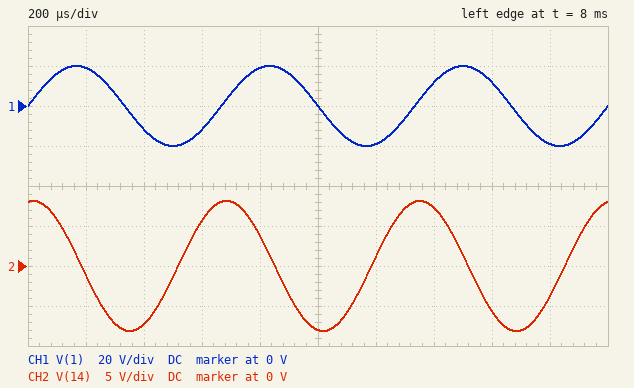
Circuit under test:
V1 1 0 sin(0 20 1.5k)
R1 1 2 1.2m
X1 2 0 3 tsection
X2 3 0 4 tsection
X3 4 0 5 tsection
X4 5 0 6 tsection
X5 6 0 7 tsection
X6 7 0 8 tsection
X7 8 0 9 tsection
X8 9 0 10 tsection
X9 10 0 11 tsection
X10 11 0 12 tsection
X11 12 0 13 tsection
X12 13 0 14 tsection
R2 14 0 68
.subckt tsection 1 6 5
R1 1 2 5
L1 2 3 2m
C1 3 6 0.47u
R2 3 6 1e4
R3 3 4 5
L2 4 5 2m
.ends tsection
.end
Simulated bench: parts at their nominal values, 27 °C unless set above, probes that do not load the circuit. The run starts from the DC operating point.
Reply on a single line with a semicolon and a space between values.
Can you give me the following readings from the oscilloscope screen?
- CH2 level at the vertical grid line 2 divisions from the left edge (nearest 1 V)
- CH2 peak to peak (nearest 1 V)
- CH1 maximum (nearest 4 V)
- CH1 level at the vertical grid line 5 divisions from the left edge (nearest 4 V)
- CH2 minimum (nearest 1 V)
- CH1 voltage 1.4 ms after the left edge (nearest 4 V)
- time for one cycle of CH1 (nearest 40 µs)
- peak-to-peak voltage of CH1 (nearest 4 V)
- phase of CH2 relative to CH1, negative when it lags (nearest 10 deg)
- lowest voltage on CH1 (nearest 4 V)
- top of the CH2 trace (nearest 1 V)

-7 V; 16 V; 20 V; 0 V; -8 V; 12 V; 680 µs; 40 V; 80 deg; -20 V; 8 V
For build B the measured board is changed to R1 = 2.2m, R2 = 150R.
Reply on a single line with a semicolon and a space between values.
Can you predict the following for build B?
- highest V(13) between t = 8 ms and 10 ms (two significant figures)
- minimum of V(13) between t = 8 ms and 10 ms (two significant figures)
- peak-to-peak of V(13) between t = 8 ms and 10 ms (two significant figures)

13 V; -13 V; 26 V
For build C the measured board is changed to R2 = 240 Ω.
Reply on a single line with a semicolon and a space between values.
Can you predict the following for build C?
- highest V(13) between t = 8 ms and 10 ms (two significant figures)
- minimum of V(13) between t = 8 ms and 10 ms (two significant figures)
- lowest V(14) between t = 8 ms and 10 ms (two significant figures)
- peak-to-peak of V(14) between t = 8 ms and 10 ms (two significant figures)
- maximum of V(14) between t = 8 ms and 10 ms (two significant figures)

15 V; -15 V; -16 V; 31 V; 16 V
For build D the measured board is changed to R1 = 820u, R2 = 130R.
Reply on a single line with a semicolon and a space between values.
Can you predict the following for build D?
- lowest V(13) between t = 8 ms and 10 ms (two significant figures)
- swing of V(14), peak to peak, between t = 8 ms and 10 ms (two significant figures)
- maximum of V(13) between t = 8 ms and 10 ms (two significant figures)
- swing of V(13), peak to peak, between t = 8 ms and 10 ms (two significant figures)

-12 V; 24 V; 12 V; 25 V
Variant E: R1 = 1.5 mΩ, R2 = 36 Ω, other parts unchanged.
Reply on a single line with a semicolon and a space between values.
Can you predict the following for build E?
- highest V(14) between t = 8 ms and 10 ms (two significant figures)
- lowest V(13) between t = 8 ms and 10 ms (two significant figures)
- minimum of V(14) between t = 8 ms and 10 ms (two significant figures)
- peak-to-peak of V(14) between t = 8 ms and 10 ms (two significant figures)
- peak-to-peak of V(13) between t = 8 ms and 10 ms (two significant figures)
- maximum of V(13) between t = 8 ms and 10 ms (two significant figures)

5.1 V; -7.9 V; -5.1 V; 10 V; 16 V; 7.9 V
